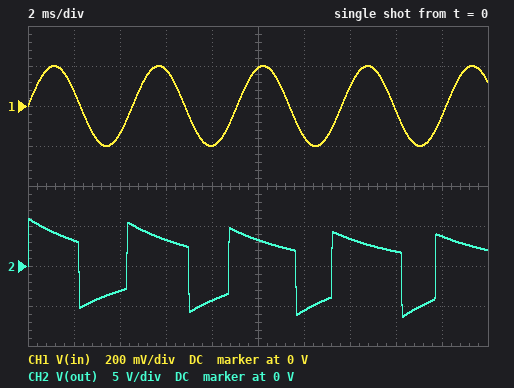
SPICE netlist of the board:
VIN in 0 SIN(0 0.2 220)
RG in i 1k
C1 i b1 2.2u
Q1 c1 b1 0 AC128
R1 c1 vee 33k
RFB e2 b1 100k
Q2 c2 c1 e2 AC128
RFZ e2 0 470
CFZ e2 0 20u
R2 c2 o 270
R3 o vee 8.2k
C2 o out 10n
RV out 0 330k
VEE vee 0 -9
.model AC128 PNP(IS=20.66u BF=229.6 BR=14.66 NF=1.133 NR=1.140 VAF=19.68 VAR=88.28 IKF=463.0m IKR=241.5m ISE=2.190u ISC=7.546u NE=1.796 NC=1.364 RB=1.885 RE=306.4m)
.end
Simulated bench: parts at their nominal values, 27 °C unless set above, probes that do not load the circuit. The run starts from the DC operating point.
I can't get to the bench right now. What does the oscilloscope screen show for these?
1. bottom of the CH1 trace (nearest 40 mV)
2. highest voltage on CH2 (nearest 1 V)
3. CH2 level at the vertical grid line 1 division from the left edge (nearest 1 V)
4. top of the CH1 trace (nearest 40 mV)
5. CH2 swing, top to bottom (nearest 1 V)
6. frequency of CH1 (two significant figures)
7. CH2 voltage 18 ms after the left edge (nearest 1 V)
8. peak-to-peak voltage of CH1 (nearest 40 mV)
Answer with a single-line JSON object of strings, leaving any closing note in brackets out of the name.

{"bottom of the CH1 trace": "-200 mV", "highest voltage on CH2": "6 V", "CH2 level at the vertical grid line 1 division from the left edge": "3 V", "top of the CH1 trace": "200 mV", "CH2 swing, top to bottom": "12 V", "frequency of CH1": "220 Hz", "CH2 voltage 18 ms after the left edge": "4 V", "peak-to-peak voltage of CH1": "400 mV"}
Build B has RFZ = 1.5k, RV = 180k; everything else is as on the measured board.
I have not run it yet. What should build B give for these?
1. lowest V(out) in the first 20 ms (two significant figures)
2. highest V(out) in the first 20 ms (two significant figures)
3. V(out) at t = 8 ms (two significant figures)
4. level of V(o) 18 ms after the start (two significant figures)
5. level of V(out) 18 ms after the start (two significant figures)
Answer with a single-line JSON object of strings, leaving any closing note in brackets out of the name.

{"lowest V(out) in the first 20 ms": "-6.7 V", "highest V(out) in the first 20 ms": "7.4 V", "V(out) at t = 8 ms": "-3.8 V", "level of V(o) 18 ms after the start": "-900 mV", "level of V(out) 18 ms after the start": "4.3 V"}
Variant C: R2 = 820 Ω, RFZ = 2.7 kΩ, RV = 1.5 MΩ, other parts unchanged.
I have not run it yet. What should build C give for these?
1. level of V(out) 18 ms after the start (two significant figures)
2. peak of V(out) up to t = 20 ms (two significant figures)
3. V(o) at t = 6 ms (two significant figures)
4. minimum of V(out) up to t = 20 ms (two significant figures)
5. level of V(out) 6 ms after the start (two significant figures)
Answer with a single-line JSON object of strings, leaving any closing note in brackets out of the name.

{"level of V(out) 18 ms after the start": "4.1 V", "peak of V(out) up to t = 20 ms": "7.3 V", "V(o) at t = 6 ms": "-1.2 V", "minimum of V(out) up to t = 20 ms": "-3.6 V", "level of V(out) 6 ms after the start": "5.7 V"}
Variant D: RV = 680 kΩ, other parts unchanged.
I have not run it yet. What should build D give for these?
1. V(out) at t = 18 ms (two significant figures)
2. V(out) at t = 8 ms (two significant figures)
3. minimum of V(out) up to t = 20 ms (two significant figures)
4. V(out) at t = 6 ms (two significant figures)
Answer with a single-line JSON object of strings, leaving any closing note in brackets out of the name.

{"V(out) at t = 18 ms": "3.5 V", "V(out) at t = 8 ms": "-4.1 V", "minimum of V(out) up to t = 20 ms": "-5.6 V", "V(out) at t = 6 ms": "4.1 V"}
